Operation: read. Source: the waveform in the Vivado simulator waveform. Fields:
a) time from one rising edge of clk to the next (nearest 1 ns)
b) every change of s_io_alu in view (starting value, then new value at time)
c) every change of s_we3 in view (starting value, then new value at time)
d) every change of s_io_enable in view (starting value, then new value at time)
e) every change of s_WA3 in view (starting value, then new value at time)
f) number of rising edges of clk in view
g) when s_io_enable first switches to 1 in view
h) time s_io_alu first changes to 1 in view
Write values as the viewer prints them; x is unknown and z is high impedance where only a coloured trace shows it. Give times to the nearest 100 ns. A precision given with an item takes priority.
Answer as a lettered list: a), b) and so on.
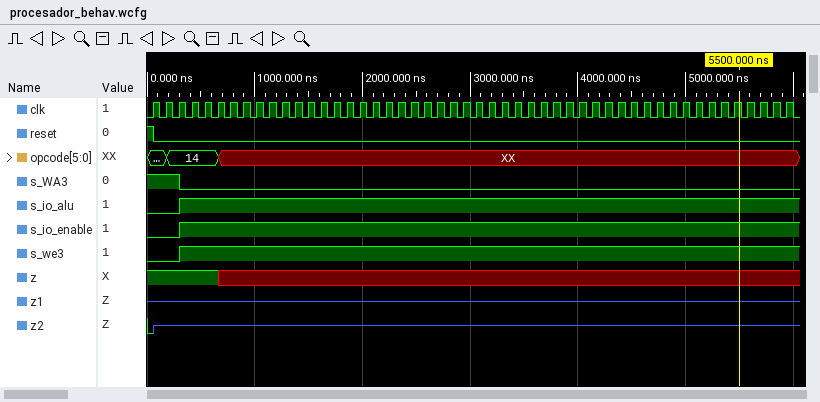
a) 120 ns
b) 0, 1 at 300 ns
c) 0, 1 at 300 ns
d) 0, 1 at 300 ns
e) 1, 0 at 300 ns
f) 50
g) 300 ns
h) 300 ns
